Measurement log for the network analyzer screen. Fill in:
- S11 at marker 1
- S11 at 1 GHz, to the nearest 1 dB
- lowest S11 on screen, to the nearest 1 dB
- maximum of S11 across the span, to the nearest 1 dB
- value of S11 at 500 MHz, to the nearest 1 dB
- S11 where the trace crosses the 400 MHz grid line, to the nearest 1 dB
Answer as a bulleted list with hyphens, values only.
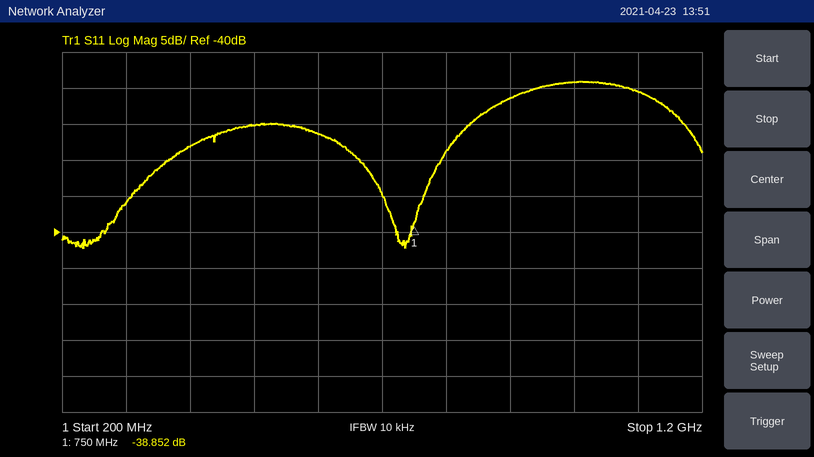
- -38.852 dB
- -19 dB
- -42 dB
- -19 dB
- -25 dB
- -28 dB
